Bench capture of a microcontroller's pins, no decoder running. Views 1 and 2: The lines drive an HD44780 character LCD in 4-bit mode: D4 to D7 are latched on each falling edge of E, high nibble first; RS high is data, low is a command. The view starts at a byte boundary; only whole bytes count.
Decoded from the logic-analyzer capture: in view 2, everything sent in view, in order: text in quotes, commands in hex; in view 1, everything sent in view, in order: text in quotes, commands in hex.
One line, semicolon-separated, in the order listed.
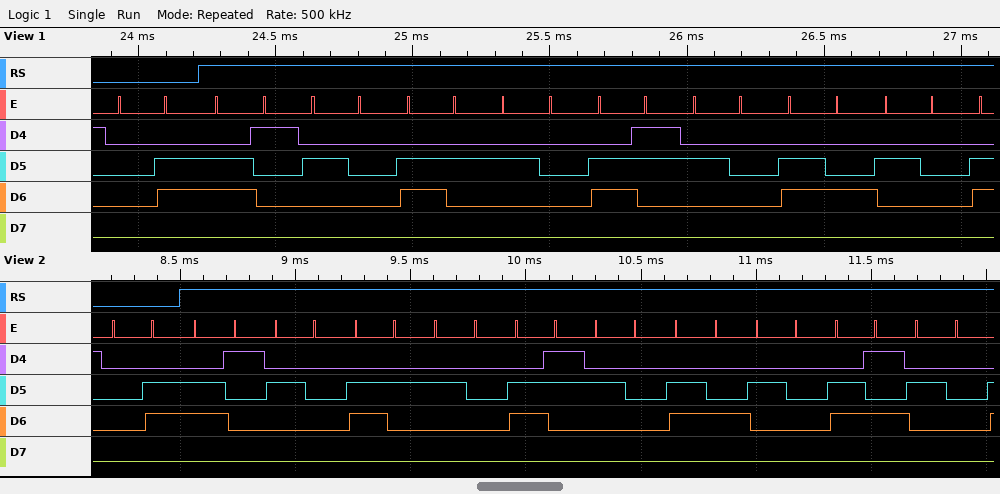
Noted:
0x06 "a b c d e "; 0x06 "a b c d "
